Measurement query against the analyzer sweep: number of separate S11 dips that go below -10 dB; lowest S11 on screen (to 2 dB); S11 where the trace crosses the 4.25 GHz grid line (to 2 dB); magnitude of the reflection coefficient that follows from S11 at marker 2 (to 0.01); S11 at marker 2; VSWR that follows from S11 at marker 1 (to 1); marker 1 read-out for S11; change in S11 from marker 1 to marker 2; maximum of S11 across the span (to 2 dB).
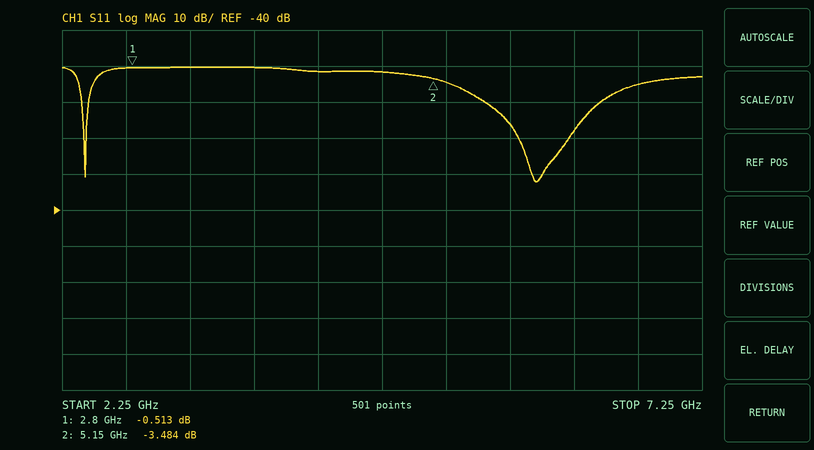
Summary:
2
-32 dB
-2 dB
0.67
-3.484 dB
34
-0.513 dB
-2.971 dB
0 dB
